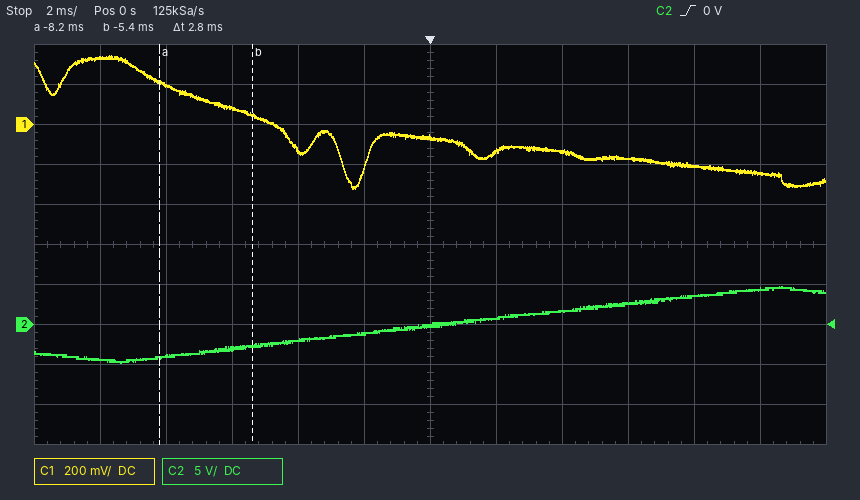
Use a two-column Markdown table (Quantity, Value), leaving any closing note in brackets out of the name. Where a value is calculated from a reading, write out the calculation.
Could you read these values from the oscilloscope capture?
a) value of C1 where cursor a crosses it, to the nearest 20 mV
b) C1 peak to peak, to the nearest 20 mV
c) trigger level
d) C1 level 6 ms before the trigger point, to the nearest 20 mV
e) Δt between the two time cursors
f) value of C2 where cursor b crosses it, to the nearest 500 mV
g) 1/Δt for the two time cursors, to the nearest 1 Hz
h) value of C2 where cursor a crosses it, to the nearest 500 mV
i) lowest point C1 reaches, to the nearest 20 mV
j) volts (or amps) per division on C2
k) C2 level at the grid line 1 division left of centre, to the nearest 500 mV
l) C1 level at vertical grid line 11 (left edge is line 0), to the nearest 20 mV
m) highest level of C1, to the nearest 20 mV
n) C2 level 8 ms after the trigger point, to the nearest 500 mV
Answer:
| Quantity | Value |
|---|---|
| value of C1 where cursor a crosses it, to the nearest 20 mV | 220 mV |
| C1 peak to peak, to the nearest 20 mV | 340 mV − (-320 mV) = 660 mV |
| trigger level | 0 V |
| C1 level 6 ms before the trigger point, to the nearest 20 mV | 80 mV |
| Δt between the two time cursors | 2.8 ms |
| value of C2 where cursor b crosses it, to the nearest 500 mV | -2.5 V |
| 1/Δt for the two time cursors, to the nearest 1 Hz | 1 / 2.8 ms ≈ 357 Hz |
| value of C2 where cursor a crosses it, to the nearest 500 mV | -4.0 V |
| lowest point C1 reaches, to the nearest 20 mV | -320 mV |
| volts (or amps) per division on C2 | 5 V |
| C2 level at the grid line 1 division left of centre, to the nearest 500 mV | -1.0 V |
| C1 level at vertical grid line 11 (left edge is line 0), to the nearest 20 mV | -240 mV |
| highest level of C1, to the nearest 20 mV | 340 mV |
| C2 level 8 ms after the trigger point, to the nearest 500 mV | 3.5 V |
